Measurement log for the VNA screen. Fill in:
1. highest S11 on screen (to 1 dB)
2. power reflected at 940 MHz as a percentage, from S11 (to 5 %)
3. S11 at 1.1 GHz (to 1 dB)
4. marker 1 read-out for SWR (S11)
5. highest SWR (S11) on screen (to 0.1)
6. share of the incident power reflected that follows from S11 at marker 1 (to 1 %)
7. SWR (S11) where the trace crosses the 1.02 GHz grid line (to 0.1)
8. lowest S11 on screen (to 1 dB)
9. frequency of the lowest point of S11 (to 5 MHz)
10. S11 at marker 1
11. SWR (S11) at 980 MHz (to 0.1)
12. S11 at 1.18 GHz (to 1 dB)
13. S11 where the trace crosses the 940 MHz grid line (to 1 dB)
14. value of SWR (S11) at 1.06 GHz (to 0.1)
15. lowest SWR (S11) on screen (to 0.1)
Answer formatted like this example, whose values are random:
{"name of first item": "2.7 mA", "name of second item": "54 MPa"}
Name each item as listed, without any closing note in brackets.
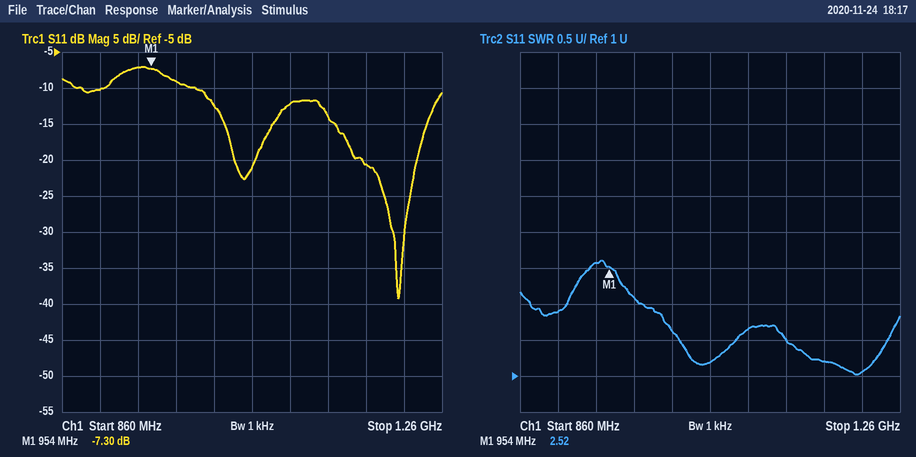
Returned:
{"highest S11 on screen": "-7 dB", "power reflected at 940 MHz as a percentage, from S11": "20 %", "S11 at 1.1 GHz": "-12 dB", "marker 1 read-out for SWR": "2.52", "highest SWR (S11) on screen": "2.6", "share of the incident power reflected that follows from S11 at marker 1": "19 %", "SWR (S11) where the trace crosses the 1.02 GHz grid line": "1.6", "lowest S11 on screen": "-39 dB", "frequency of the lowest point of S11": "1.215 GHz", "S11 at marker 1": "-7.30 dB", "SWR (S11) at 980 MHz": "2.1", "S11 at 1.18 GHz": "-21 dB", "S11 where the trace crosses the 940 MHz grid line": "-7 dB", "value of SWR (S11) at 1.06 GHz": "1.2", "lowest SWR (S11) on screen": "1.0"}
